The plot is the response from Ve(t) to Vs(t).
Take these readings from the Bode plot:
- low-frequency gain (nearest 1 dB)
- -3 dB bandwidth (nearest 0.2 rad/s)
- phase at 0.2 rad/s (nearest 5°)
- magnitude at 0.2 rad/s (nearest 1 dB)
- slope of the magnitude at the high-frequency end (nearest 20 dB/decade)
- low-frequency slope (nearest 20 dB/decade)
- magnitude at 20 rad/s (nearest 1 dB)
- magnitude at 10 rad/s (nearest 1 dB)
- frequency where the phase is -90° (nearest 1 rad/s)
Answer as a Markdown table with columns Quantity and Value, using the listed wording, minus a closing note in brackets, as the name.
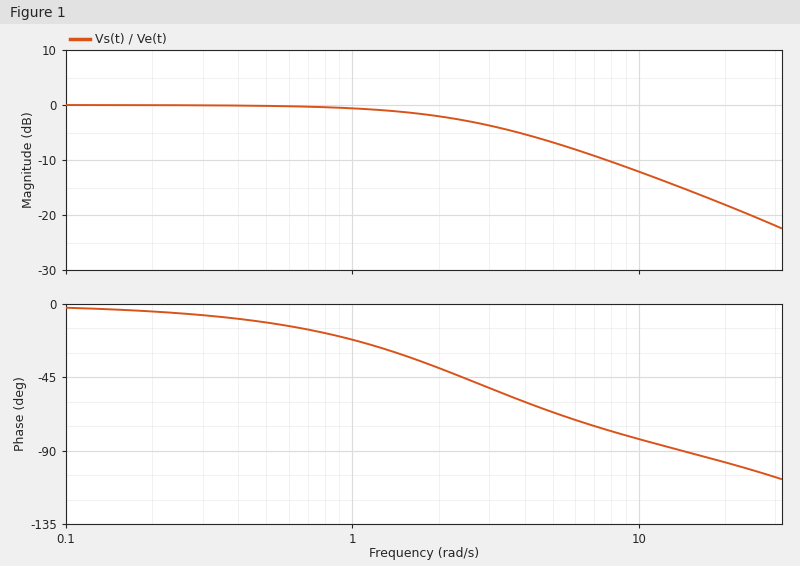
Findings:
| Quantity | Value |
|---|---|
| low-frequency gain | 0 dB |
| -3 dB bandwidth | 2.6 rad/s |
| phase at 0.2 rad/s | -5° |
| magnitude at 0.2 rad/s | 0 dB |
| slope of the magnitude at the high-frequency end | -20 dB/decade |
| low-frequency slope | 0 dB/decade |
| magnitude at 20 rad/s | -18 dB |
| magnitude at 10 rad/s | -12 dB |
| frequency where the phase is -90° | 14 rad/s |
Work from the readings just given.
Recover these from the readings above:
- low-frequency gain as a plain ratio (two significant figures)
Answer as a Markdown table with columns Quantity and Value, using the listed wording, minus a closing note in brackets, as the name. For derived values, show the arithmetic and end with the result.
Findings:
| Quantity | Value |
|---|---|
| low-frequency gain as a plain ratio | 10^(0 / 20) = 1.0 |
